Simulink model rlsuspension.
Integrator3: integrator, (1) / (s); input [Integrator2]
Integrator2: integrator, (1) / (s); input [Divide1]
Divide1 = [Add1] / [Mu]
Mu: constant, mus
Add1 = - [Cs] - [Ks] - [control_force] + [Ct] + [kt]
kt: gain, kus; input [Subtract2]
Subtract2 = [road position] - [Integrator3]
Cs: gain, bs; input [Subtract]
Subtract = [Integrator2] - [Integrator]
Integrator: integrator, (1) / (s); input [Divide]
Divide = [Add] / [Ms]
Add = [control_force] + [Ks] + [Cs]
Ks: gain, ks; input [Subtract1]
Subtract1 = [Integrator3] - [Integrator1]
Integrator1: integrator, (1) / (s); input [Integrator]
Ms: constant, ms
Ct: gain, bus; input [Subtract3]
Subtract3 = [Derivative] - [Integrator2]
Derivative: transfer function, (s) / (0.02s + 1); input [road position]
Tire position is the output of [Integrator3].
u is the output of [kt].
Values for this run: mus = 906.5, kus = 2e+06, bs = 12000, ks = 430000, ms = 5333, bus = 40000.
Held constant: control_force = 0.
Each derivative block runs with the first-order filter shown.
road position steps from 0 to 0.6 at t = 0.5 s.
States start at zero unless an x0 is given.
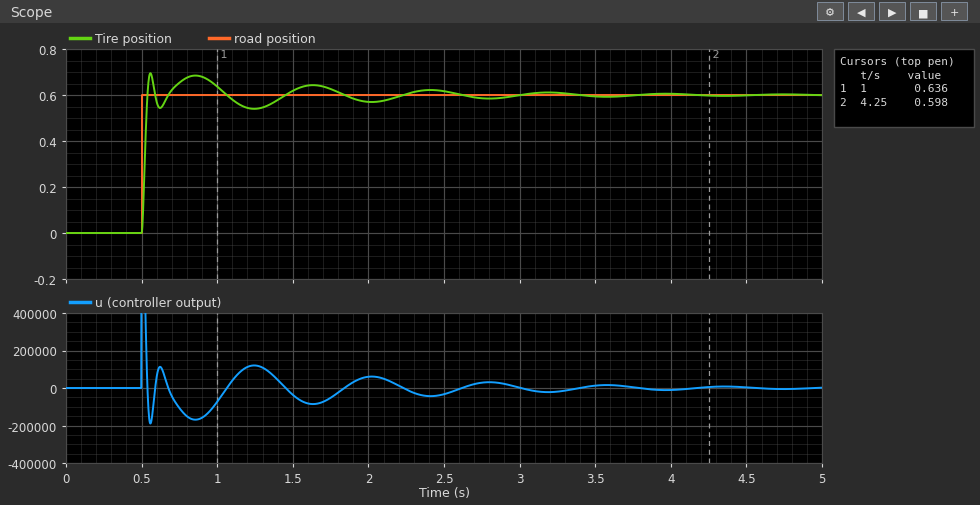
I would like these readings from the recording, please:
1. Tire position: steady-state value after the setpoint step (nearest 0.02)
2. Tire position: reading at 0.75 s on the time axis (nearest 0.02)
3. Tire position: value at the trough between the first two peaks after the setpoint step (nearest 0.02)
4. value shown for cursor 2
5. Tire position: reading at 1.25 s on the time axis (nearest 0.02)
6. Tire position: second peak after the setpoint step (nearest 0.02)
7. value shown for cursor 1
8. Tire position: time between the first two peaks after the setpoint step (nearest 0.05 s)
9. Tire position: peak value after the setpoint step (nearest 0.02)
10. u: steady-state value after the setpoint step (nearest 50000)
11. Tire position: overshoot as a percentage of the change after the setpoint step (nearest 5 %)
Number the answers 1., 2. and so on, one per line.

1. 0.60
2. 0.66
3. 0.54
4. 0.598
5. 0.54
6. 0.68
7. 0.636
8. 0.30 s
9. 0.70
10. 0
11. 15 %
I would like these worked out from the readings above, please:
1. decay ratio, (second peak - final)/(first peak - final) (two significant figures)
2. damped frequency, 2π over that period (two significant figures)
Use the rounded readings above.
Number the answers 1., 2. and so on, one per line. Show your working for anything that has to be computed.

1. (0.68 - 0.6) / (0.7 - 0.6) = 0.80
2. 2π / 0.3 = 21 rad/s
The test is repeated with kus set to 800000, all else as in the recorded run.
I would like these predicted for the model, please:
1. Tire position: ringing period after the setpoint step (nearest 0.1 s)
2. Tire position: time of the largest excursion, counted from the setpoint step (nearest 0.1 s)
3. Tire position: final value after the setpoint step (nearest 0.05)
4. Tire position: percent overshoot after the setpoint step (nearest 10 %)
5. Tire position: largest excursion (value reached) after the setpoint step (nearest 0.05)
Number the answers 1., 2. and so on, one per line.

1. 0.9 s
2. 0.4 s
3. 0.60
4. 30 %
5. 0.75
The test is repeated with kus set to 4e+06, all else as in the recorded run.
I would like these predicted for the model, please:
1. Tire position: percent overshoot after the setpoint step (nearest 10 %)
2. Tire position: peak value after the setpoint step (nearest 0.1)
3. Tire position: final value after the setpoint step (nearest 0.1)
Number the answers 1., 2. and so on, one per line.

1. 30 %
2. 0.8
3. 0.6
